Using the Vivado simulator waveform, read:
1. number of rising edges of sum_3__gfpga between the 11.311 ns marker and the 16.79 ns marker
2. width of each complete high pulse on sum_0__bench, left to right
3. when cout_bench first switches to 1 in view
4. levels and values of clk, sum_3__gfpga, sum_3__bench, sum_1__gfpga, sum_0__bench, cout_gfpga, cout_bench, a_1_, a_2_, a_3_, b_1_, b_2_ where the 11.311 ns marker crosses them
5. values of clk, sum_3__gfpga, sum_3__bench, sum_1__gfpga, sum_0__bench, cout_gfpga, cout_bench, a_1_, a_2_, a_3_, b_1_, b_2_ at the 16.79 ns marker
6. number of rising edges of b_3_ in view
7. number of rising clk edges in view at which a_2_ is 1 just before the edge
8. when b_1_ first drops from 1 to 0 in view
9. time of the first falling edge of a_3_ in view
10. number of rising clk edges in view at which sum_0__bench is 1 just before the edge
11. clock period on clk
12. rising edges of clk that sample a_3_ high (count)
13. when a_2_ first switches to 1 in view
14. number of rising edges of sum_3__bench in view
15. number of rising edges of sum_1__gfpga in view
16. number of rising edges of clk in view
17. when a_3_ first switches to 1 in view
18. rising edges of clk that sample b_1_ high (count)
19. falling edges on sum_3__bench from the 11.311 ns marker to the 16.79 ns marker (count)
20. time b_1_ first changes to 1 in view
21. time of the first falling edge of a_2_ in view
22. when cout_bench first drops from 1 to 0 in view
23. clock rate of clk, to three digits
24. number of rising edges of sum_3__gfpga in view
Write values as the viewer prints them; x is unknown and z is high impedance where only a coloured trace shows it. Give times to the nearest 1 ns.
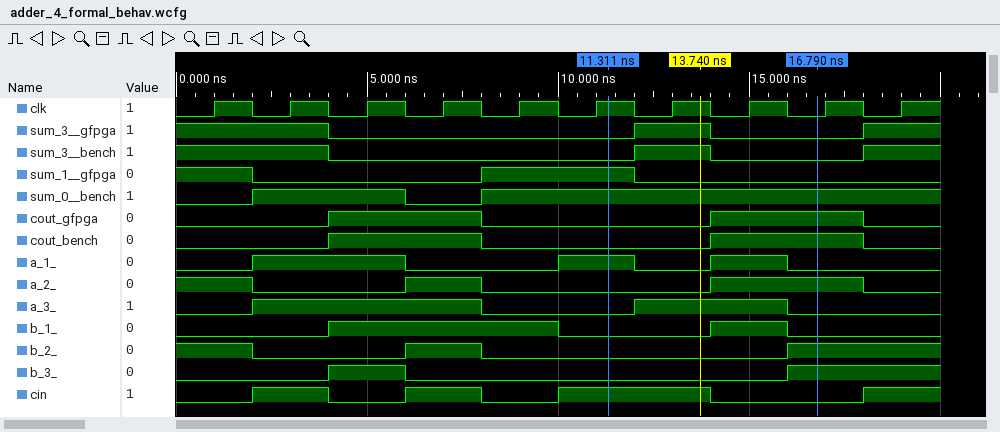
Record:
1
4 ns
4 ns
clk=1, sum_3__gfpga=0, sum_3__bench=0, sum_1__gfpga=1, sum_0__bench=1, cout_gfpga=0, cout_bench=0, a_1_=1, a_2_=0, a_3_=0, b_1_=0, b_2_=0
clk=0, sum_3__gfpga=0, sum_3__bench=0, sum_1__gfpga=0, sum_0__bench=1, cout_gfpga=1, cout_bench=1, a_1_=0, a_2_=1, a_3_=0, b_1_=0, b_2_=1
2
4
10 ns
8 ns
8
2 ns
5
6 ns
2
1
10
2 ns
4
1
4 ns
2 ns
8 ns
500 MHz
2
